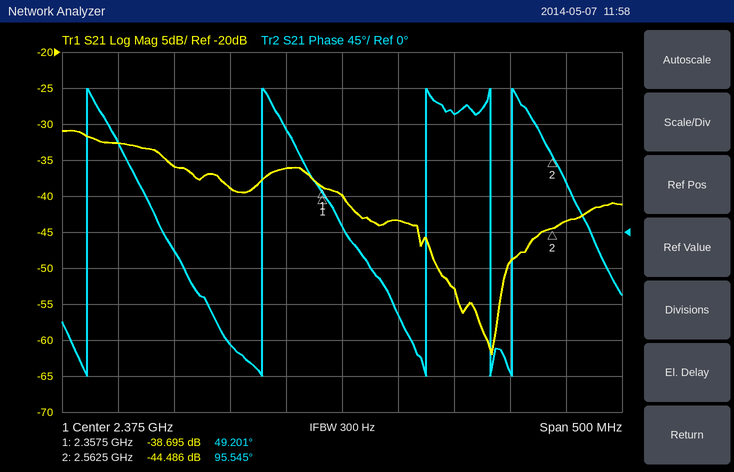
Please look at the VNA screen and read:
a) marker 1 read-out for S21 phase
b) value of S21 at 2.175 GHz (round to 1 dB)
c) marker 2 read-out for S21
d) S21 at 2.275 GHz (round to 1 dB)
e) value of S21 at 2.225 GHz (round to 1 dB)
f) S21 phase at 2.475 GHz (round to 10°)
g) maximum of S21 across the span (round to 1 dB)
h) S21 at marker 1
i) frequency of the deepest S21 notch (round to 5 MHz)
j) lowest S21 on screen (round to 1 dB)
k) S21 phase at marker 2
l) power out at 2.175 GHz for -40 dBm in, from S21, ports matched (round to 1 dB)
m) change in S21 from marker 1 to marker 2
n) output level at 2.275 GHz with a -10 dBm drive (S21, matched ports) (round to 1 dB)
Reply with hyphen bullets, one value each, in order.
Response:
- 49.201°
- -33 dB
- -44.486 dB
- -39 dB
- -36 dB
- 150°
- -31 dB
- -38.695 dB
- 2.510 GHz
- -62 dB
- 95.545°
- -73 dBm
- -5.791 dB
- -49 dBm
